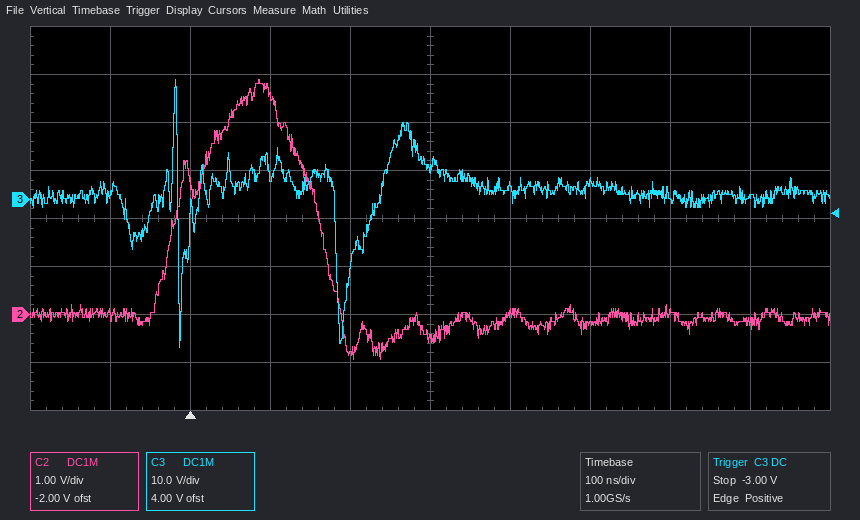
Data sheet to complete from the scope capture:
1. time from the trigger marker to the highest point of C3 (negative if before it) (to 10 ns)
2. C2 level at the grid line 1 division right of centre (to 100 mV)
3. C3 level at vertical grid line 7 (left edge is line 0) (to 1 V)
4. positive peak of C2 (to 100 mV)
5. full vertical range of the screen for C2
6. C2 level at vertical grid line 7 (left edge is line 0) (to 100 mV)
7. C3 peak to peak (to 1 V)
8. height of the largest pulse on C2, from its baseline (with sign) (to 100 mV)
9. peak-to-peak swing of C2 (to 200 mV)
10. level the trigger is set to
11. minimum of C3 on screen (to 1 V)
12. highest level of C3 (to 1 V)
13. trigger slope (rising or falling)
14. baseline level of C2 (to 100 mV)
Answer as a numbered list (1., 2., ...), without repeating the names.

1. -20 ns
2. 0.0 V
3. 4 V
4. 4.9 V
5. 8 V
6. -200 mV
7. 56 V
8. +4.9 V
9. 5.8 V
10. -3.00 V
11. -31 V
12. 25 V
13. rising
14. 0.0 V
